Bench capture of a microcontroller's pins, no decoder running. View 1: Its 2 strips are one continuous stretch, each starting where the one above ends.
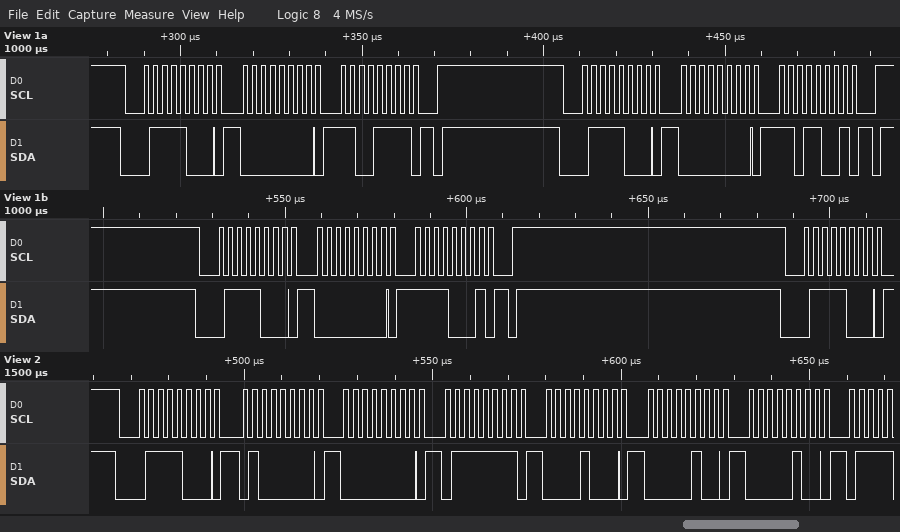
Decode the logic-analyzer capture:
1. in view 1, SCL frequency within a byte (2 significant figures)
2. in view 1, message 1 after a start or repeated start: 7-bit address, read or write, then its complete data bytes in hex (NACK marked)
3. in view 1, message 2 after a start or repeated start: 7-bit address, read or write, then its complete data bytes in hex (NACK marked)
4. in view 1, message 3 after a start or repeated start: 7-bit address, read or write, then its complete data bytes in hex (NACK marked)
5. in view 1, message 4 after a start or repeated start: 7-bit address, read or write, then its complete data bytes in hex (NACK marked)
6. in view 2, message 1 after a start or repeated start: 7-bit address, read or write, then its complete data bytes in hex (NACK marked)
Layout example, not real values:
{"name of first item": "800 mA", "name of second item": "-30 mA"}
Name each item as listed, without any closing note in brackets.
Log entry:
{"in view 1, SCL frequency within a byte": "400 kHz", "in view 1, message 1 after a start or repeated start: 7-bit address, read or write, then its complete data bytes in hex": "0x3C write: 00 CF", "in view 1, message 2 after a start or repeated start: 7-bit address, read or write, then its complete data bytes in hex": "0x3C write: 00 D9", "in view 1, message 3 after a start or repeated start: 7-bit address, read or write, then its complete data bytes in hex": "0x3C write: 00 F1", "in view 1, message 4 after a start or repeated start: 7-bit address, read or write, then its complete data bytes in hex": "0x3C write", "in view 2, message 1 after a start or repeated start: 7-bit address, read or write, then its complete data bytes in hex": "0x3C write: 40 00 7F 08 04 04"}
